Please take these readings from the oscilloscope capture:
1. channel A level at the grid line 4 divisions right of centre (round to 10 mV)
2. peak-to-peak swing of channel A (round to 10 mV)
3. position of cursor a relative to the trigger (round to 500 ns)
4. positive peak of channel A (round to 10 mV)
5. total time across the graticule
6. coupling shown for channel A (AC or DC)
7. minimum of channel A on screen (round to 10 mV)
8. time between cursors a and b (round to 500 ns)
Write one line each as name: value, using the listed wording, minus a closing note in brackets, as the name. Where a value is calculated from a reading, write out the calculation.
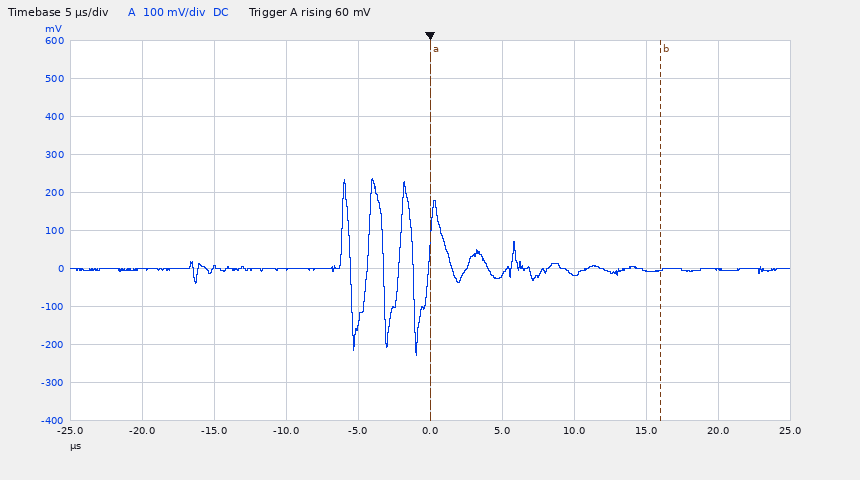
channel A level at the grid line 4 divisions right of centre: 0 mV
peak-to-peak swing of channel A: 240 mV − (-230 mV) = 470 mV
position of cursor a relative to the trigger: 0.0 µs
positive peak of channel A: 240 mV
total time across the graticule: 50 µs
coupling shown for channel A: DC
minimum of channel A on screen: -230 mV
time between cursors a and b: 16.0 µs
